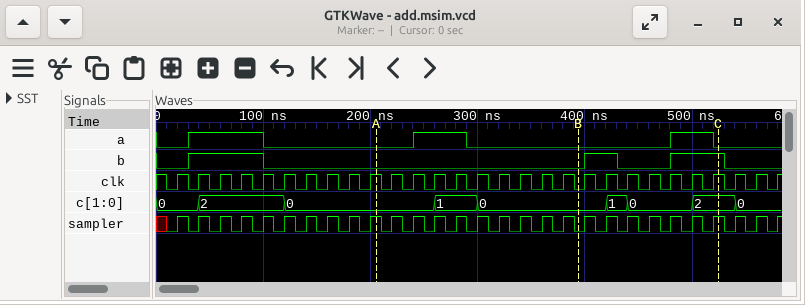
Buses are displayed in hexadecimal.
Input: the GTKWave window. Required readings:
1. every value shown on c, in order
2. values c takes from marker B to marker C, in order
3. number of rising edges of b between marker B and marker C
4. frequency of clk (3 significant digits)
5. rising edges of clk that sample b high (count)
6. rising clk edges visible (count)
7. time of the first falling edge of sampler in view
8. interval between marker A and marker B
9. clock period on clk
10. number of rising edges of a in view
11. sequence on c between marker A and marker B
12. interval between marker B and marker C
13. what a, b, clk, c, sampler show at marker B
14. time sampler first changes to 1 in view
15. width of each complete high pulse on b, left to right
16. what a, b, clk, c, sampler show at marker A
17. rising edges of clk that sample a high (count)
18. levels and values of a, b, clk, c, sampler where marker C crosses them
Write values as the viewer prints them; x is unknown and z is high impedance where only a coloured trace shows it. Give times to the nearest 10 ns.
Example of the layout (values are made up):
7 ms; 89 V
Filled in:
0, 2, 0, 1, 0, 1, 0, 2, 0; 0, 1, 0, 2; 2; 50.0 MHz; 7; 29; 30 ns; 190 ns; 20 ns; 3; 0, 1, 0; 130 ns; a=0, b=0, clk=0, c=0, sampler=0; 20 ns; 70 ns, 30 ns, 50 ns; a=0, b=0, clk=1, c=0, sampler=1; 8; a=0, b=1, clk=1, c=2, sampler=1
